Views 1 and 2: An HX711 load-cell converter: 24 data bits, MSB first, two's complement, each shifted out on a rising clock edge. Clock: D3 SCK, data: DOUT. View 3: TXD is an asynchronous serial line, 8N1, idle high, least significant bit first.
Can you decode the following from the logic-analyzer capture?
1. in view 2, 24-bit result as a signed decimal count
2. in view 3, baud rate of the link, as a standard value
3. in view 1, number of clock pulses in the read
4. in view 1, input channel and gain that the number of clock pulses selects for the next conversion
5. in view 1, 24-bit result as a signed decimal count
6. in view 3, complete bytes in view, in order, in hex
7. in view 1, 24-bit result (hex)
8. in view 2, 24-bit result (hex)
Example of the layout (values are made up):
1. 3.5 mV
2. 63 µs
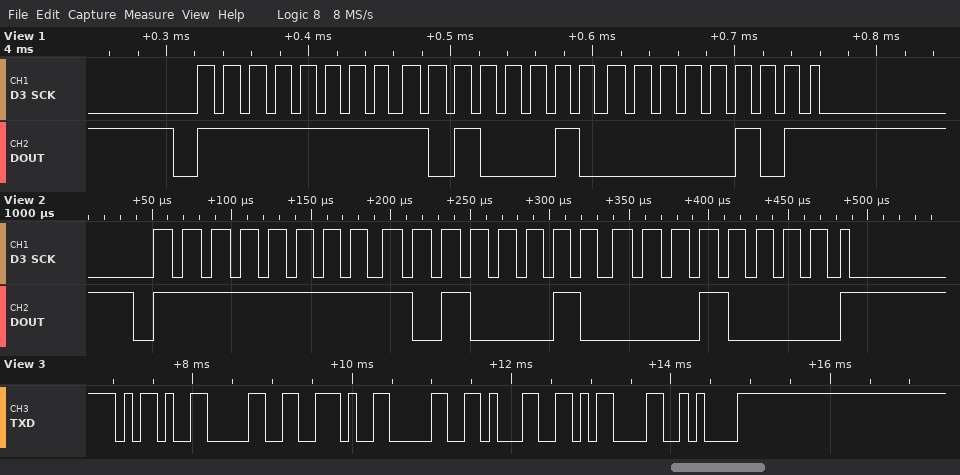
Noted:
1. -24048
2. 9600 baud
3. 25
4. channel A, gain 128
5. -24059
6. 0x2D 0x30 0x2E 0x30 0x31 0x0D 0x0A
7. 0xFFA205
8. 0xFFA210
